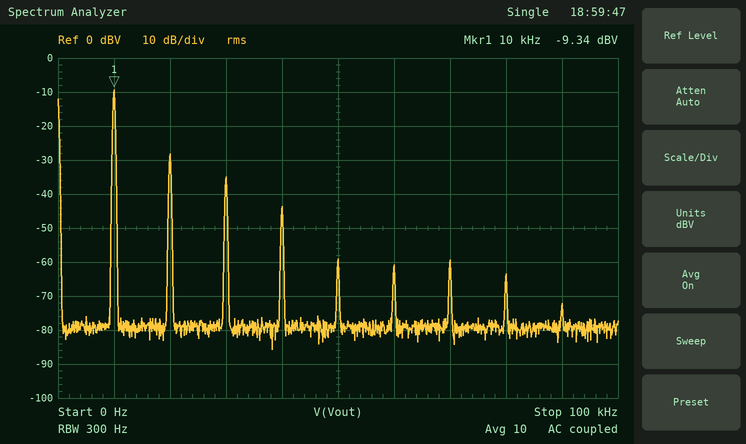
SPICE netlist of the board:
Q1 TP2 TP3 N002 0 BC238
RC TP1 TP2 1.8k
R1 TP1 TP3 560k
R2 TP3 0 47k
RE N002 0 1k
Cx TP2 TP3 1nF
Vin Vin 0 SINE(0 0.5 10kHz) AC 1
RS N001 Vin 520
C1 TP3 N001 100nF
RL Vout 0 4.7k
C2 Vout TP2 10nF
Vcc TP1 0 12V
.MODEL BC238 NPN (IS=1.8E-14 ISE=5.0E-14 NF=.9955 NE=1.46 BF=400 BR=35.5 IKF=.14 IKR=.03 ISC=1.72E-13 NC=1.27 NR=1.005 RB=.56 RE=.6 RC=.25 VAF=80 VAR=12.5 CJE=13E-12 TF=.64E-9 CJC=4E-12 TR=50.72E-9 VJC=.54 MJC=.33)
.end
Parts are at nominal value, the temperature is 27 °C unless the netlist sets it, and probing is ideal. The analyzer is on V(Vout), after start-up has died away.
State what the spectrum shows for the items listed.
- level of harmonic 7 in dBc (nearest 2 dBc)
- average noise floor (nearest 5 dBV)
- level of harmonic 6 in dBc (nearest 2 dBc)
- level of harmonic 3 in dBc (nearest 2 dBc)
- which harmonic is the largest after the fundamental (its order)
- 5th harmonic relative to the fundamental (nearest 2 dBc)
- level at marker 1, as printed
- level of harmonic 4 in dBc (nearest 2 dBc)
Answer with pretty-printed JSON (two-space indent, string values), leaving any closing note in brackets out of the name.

{
  "level of harmonic 7 in dBc": "-50 dBc",
  "average noise floor": "-80 dBV",
  "level of harmonic 6 in dBc": "-52 dBc",
  "level of harmonic 3 in dBc": "-26 dBc",
  "which harmonic is the largest after the fundamental": "2",
  "5th harmonic relative to the fundamental": "-50 dBc",
  "level at marker 1, as printed": "-9.34 dBV",
  "level of harmonic 4 in dBc": "-34 dBc"
}
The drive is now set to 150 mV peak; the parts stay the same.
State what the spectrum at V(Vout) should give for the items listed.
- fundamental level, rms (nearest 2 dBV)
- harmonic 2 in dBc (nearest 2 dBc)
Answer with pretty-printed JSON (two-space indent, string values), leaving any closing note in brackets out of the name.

{
  "fundamental level, rms": "-18 dBV",
  "harmonic 2 in dBc": "-40 dBc"
}
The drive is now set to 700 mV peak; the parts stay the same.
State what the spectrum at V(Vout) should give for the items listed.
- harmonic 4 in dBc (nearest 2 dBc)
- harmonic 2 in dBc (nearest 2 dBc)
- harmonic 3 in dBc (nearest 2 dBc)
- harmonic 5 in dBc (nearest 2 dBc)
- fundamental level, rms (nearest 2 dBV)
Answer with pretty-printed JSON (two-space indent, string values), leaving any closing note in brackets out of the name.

{
  "harmonic 4 in dBc": "-44 dBc",
  "harmonic 2 in dBc": "-14 dBc",
  "harmonic 3 in dBc": "-22 dBc",
  "harmonic 5 in dBc": "-36 dBc",
  "fundamental level, rms": "-8 dBV"
}
